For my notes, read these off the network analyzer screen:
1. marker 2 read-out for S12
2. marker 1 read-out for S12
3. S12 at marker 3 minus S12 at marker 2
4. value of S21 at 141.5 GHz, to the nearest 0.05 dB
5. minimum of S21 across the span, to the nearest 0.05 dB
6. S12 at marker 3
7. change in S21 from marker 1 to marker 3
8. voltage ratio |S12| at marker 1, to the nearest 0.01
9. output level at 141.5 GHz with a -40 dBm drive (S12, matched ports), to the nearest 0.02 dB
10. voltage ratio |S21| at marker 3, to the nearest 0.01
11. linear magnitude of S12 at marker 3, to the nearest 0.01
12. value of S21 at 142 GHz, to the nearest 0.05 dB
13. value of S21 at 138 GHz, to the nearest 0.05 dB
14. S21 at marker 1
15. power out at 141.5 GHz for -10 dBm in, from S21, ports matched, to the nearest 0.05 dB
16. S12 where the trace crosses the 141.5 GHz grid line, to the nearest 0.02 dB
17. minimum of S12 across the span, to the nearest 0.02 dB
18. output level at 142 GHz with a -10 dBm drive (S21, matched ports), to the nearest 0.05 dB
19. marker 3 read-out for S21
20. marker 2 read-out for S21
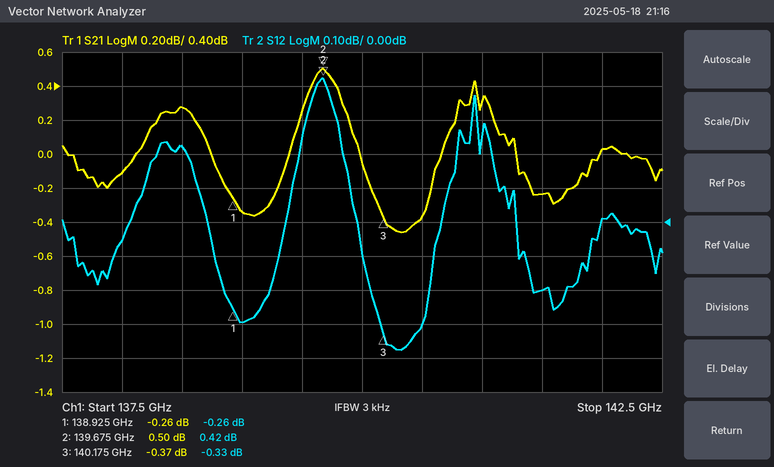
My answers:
0.42 dB
-0.26 dB
-0.75 dB
-0.25 dB
-0.45 dB
-0.33 dB
-0.11 dB
0.97
-40.20 dBm
0.96
0.96
0.05 dB
-0.10 dB
-0.26 dB
-10.25 dBm
-0.20 dB
-0.38 dB
-9.95 dBm
-0.37 dB
0.50 dB
